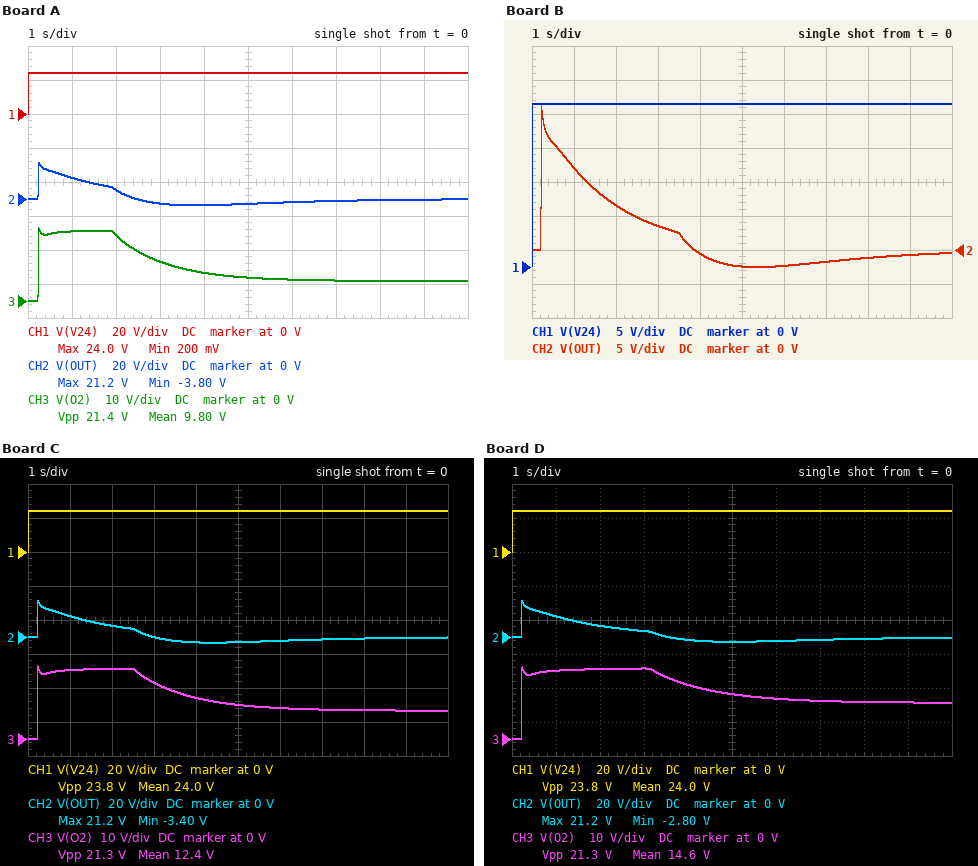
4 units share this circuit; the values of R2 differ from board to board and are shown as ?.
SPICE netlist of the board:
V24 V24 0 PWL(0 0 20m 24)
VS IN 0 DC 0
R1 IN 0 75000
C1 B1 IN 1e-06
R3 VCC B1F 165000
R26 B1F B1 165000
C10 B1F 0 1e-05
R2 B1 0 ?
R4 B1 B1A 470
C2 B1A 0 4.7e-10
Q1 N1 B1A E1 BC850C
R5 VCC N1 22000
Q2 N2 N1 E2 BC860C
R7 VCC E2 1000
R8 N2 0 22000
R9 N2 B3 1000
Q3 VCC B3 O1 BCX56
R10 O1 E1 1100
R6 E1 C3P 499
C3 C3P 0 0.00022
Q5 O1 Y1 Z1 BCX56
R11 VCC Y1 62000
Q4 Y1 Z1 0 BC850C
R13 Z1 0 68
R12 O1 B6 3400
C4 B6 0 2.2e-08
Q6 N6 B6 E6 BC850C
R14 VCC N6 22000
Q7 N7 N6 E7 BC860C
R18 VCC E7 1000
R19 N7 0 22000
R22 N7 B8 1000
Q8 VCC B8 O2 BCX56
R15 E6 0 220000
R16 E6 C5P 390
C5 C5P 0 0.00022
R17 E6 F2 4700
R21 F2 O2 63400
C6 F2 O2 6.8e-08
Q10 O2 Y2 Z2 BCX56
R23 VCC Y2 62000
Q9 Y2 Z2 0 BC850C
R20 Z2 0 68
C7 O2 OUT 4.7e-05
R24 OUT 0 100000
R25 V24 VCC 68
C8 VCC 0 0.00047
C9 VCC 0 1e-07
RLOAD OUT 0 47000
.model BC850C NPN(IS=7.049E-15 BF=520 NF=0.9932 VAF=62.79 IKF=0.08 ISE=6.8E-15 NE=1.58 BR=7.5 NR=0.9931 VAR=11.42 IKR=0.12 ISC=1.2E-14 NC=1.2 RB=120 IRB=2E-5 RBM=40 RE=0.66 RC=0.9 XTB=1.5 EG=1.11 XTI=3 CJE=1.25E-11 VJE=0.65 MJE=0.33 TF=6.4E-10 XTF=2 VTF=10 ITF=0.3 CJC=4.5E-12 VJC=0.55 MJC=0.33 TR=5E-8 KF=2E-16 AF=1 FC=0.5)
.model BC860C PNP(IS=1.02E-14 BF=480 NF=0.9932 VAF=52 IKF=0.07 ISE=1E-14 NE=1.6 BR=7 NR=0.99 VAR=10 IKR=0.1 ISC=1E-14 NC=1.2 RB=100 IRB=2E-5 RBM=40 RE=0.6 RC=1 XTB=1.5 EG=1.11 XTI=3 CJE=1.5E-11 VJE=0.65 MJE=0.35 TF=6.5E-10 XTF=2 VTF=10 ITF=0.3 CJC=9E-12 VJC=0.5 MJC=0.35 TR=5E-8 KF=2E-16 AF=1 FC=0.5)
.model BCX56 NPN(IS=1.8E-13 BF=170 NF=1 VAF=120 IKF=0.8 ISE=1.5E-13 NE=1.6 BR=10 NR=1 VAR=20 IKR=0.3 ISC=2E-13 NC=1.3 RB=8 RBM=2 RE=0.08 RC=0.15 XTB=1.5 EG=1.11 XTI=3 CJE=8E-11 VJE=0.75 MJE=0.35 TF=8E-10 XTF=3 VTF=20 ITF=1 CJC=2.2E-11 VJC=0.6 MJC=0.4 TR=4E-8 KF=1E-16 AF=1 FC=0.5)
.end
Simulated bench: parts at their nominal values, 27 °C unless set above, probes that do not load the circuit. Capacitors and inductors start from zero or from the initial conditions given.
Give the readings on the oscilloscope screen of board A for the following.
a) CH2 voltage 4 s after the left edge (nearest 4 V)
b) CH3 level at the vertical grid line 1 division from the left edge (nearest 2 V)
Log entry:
-4 V
20 V
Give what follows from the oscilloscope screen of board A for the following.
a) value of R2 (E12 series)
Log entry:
180 kΩ
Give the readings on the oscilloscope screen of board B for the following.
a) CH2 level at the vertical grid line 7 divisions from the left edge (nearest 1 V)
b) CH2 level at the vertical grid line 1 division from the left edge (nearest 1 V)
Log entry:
-2 V
12 V
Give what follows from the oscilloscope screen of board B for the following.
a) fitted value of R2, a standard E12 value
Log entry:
470 kΩ
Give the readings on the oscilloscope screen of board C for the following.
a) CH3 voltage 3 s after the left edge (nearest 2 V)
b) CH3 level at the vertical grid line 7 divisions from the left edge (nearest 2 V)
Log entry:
16 V
8 V
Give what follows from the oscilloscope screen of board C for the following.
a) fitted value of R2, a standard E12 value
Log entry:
270 kΩ
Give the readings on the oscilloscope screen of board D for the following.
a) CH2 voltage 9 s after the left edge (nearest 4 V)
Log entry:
0 V
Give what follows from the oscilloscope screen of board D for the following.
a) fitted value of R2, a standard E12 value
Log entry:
390 kΩ
